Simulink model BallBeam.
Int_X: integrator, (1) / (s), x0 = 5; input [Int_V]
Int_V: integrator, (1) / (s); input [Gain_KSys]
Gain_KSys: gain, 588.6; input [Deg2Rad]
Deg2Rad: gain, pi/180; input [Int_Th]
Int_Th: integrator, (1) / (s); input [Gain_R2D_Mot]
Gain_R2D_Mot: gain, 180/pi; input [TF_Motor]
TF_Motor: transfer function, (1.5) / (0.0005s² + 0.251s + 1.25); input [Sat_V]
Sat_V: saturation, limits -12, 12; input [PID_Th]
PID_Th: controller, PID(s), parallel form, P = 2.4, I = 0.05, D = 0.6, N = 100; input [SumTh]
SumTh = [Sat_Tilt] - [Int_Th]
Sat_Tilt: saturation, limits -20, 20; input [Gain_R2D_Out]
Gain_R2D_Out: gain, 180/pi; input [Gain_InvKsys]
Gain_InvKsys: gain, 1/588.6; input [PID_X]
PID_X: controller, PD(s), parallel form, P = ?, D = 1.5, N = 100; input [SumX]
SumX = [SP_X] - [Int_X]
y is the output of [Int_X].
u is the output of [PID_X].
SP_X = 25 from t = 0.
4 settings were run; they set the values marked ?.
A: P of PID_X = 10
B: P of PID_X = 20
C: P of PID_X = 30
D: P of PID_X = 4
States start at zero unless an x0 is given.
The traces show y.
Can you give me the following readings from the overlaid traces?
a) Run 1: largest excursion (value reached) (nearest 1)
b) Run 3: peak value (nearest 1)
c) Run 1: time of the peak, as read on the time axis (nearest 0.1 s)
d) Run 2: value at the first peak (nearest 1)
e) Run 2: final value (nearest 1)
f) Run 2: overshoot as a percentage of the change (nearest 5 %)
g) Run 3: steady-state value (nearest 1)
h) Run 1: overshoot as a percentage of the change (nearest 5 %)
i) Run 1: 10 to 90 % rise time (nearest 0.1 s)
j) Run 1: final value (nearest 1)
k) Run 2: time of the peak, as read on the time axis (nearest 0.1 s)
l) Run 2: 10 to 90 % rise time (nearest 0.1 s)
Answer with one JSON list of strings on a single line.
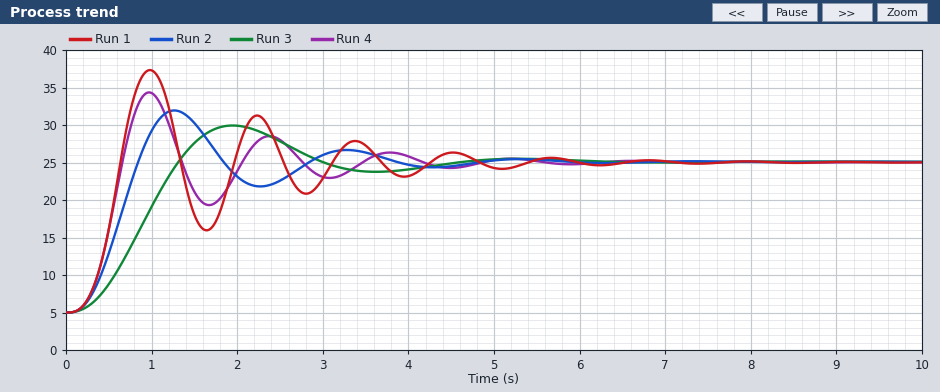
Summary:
["37", "30", "1.0 s", "32", "25", "35 %", "25", "60 %", "0.3 s", "25", "1.3 s", "0.5 s"]
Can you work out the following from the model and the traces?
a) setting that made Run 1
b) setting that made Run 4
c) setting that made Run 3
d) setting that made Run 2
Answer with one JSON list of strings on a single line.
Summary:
["C", "B", "D", "A"]
